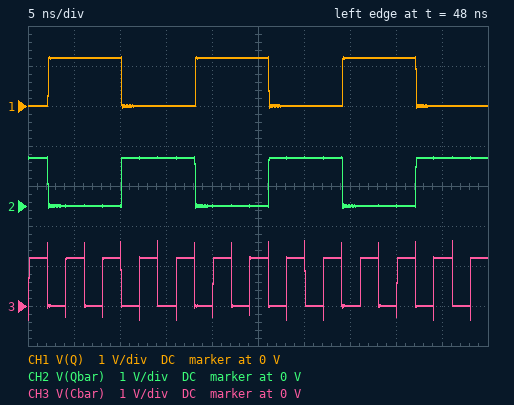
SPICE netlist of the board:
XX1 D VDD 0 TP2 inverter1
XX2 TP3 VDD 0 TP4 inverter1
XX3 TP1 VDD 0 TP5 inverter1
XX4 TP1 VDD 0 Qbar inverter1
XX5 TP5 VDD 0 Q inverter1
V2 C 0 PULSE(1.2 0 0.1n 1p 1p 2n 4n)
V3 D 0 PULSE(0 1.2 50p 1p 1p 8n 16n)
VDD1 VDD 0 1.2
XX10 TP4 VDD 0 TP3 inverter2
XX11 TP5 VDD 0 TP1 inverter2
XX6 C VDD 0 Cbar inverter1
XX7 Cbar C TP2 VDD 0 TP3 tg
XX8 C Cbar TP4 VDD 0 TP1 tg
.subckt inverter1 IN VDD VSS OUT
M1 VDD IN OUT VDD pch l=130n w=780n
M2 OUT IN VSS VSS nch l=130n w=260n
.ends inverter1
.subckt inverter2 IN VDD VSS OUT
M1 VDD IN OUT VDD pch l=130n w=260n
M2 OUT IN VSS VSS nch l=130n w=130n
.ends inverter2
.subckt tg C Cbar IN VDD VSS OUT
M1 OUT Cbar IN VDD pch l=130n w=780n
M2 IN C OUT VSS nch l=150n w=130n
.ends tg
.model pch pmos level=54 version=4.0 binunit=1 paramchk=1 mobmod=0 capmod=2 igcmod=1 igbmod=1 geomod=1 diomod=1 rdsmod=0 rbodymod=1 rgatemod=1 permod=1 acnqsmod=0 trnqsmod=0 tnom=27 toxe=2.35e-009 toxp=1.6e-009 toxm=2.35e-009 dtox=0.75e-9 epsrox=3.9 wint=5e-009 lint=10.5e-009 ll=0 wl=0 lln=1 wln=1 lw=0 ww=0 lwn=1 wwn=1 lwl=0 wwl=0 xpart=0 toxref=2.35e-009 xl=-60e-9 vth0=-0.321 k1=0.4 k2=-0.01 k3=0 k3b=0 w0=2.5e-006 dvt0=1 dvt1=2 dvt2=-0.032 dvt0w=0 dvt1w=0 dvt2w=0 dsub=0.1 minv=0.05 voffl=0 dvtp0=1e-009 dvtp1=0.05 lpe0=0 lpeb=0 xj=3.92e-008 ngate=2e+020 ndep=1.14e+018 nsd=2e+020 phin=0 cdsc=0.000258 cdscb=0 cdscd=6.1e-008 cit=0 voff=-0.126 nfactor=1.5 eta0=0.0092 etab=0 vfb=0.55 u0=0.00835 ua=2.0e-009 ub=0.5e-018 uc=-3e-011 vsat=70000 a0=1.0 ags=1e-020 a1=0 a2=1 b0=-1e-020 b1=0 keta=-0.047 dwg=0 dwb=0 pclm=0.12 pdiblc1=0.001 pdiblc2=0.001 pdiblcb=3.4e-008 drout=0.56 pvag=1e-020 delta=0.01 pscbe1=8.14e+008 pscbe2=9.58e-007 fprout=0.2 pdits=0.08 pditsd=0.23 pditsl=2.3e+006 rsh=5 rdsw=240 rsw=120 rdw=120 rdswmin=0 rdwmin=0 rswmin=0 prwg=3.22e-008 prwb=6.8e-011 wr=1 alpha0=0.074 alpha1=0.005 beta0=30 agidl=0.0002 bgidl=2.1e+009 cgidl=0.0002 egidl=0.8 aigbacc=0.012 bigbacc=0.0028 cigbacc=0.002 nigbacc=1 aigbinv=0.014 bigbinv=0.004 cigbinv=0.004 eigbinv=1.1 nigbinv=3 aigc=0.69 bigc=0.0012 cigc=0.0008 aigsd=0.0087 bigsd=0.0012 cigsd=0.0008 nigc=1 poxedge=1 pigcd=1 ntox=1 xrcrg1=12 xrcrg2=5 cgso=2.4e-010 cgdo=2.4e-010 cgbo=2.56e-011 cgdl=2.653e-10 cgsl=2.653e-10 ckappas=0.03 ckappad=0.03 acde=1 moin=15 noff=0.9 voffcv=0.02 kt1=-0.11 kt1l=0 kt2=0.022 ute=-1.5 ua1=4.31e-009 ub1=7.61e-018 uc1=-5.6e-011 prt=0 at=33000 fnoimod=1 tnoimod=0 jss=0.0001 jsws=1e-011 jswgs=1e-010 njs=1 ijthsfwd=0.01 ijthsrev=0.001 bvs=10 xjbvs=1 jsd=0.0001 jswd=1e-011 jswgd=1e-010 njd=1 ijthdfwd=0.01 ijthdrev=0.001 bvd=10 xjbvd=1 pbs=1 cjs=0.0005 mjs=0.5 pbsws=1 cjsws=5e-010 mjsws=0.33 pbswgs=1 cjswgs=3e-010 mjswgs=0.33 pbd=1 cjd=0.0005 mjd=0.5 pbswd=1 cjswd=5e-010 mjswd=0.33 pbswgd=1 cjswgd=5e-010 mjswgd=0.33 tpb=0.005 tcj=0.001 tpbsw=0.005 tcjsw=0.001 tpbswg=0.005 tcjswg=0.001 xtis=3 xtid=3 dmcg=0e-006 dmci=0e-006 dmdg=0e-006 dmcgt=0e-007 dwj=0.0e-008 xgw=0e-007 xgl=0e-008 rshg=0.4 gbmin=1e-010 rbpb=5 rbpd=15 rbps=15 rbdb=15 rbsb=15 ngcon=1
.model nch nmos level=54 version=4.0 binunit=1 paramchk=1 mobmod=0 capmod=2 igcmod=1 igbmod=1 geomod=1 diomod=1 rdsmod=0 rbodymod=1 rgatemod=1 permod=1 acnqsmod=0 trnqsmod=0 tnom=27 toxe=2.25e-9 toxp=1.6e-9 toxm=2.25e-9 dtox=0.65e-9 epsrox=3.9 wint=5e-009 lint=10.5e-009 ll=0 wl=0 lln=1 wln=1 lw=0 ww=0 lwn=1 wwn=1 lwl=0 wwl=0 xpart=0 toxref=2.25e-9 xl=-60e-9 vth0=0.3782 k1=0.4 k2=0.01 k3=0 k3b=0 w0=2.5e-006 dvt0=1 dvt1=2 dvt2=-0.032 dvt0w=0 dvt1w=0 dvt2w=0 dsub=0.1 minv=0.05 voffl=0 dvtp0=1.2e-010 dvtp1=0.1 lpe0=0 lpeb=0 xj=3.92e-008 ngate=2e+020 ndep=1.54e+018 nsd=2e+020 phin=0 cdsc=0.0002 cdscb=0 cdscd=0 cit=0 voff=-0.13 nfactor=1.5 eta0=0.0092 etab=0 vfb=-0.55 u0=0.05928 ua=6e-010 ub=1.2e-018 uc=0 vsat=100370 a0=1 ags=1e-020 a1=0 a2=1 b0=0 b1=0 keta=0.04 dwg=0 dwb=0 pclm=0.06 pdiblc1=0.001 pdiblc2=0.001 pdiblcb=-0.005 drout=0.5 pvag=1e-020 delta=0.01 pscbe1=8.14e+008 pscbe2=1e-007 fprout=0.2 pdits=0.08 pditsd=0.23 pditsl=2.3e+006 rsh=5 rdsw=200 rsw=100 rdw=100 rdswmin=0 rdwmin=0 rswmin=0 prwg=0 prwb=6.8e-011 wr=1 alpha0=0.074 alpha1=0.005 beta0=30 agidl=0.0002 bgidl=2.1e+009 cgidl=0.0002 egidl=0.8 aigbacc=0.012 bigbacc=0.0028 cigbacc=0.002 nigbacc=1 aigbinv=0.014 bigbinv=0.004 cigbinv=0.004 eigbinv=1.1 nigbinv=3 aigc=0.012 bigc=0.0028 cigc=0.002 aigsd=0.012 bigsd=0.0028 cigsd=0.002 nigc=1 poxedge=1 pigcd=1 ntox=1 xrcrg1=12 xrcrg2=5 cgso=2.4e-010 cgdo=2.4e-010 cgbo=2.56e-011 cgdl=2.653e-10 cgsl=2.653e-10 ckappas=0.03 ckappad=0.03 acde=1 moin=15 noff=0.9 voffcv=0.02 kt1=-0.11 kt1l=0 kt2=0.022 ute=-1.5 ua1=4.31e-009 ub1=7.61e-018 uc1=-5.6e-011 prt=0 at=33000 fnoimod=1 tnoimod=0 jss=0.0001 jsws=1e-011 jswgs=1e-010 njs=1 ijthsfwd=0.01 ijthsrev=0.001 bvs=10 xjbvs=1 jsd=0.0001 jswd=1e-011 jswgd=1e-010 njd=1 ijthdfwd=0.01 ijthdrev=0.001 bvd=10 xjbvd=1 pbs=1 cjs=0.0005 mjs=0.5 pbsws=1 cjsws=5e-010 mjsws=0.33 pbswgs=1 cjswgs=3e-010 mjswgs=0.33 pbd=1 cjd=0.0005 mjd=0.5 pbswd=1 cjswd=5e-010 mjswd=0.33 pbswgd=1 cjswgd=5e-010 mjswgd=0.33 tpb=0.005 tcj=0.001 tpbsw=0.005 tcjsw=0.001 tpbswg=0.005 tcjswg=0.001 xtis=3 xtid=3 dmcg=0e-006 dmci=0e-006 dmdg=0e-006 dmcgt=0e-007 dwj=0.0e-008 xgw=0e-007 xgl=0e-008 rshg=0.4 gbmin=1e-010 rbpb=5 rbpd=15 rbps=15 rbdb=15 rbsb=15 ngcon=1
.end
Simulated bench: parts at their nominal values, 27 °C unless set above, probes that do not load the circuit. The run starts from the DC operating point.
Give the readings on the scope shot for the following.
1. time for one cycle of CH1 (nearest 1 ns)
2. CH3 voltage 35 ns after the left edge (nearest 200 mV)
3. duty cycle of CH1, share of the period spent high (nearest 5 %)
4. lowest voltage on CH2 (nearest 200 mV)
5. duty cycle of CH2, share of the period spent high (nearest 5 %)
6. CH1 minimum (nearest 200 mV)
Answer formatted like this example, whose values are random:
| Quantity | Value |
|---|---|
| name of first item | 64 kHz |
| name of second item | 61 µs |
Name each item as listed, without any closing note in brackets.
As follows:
| Quantity | Value |
|---|---|
| time for one cycle of CH1 | 16 ns |
| CH3 voltage 35 ns after the left edge | 0 V |
| duty cycle of CH1, share of the period spent high | 50 % |
| lowest voltage on CH2 | 0 V |
| duty cycle of CH2, share of the period spent high | 50 % |
| CH1 minimum | 0 V |
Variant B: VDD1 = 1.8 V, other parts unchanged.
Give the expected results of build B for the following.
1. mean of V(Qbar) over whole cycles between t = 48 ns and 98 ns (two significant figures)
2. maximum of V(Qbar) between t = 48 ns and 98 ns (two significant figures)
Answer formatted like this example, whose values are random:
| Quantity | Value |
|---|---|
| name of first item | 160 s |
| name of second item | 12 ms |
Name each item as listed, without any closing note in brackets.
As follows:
| Quantity | Value |
|---|---|
| mean of V(Qbar) over whole cycles between t = 48 ns and 98 ns | 900 mV |
| maximum of V(Qbar) between t = 48 ns and 98 ns | 1.8 V |
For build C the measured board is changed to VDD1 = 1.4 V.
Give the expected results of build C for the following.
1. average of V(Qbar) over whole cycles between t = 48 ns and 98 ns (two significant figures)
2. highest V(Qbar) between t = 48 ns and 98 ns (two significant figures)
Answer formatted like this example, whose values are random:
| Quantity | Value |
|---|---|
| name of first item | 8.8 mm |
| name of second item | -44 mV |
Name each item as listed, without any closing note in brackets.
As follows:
| Quantity | Value |
|---|---|
| average of V(Qbar) over whole cycles between t = 48 ns and 98 ns | 700 mV |
| highest V(Qbar) between t = 48 ns and 98 ns | 1.4 V |
